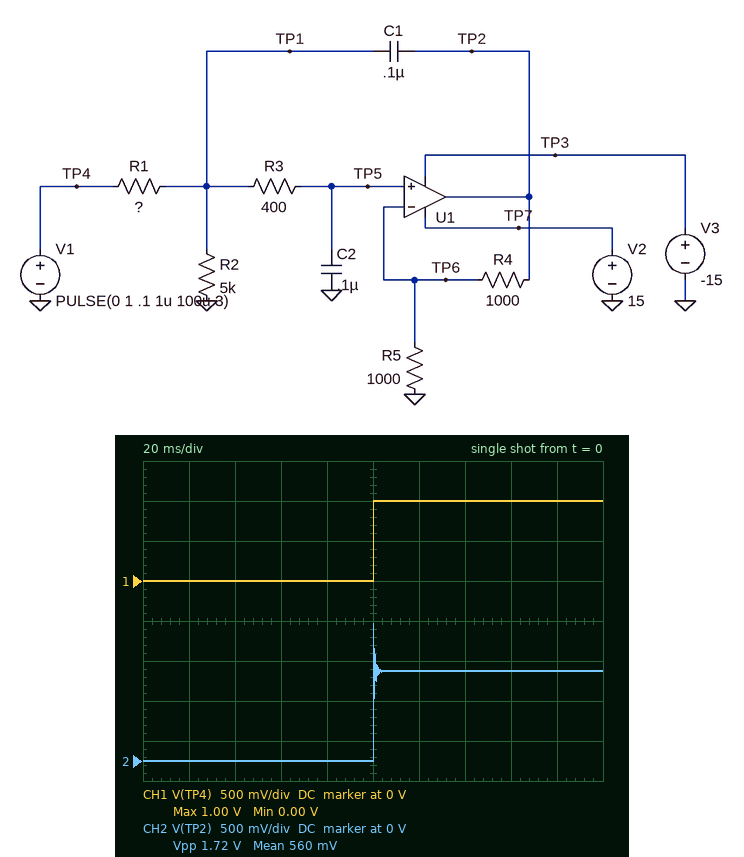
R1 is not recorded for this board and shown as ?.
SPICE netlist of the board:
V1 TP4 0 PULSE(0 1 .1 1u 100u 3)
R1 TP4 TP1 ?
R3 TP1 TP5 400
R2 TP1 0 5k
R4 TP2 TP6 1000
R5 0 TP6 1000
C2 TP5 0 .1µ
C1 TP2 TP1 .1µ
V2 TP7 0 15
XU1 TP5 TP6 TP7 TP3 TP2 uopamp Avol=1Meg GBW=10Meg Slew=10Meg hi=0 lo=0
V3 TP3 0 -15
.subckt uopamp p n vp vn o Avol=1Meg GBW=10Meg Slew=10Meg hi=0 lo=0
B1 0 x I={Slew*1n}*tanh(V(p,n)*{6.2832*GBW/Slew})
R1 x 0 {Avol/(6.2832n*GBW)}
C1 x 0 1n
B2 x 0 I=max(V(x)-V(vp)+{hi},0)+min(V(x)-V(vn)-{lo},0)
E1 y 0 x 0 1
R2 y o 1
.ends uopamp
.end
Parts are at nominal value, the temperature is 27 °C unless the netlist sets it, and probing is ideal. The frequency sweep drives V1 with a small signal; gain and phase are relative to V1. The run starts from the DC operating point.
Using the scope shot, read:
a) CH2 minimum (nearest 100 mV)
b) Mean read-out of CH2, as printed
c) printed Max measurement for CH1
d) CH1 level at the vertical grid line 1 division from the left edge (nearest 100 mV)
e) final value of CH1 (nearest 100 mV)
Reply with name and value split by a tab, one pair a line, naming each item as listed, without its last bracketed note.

CH2 minimum	0 V
Mean read-out of CH2, as printed	560 mV
printed Max measurement for CH1	1.00 V
CH1 level at the vertical grid line 1 division from the left edge	0 V
final value of CH1	1.0 V
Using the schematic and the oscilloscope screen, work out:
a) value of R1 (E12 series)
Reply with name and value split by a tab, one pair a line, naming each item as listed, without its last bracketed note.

value of R1	3.9 kΩ
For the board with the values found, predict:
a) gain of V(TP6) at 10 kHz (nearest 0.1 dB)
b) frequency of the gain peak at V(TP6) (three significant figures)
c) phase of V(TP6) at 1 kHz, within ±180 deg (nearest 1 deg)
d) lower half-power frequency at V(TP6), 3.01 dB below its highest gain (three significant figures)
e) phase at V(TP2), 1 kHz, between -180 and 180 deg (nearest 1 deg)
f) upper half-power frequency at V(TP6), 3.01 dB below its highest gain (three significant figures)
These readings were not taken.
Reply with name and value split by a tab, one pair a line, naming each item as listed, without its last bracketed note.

gain of V(TP6) at 10 kHz	-35.6 dB
frequency of the gain peak at V(TP6)	1.62 kHz
phase of V(TP6) at 1 kHz, within ±180 deg	-21 deg
lower half-power frequency at V(TP6), 3.01 dB below its highest gain	1.19 kHz
phase at V(TP2), 1 kHz, between -180 and 180 deg	-21 deg
upper half-power frequency at V(TP6), 3.01 dB below its highest gain	1.96 kHz
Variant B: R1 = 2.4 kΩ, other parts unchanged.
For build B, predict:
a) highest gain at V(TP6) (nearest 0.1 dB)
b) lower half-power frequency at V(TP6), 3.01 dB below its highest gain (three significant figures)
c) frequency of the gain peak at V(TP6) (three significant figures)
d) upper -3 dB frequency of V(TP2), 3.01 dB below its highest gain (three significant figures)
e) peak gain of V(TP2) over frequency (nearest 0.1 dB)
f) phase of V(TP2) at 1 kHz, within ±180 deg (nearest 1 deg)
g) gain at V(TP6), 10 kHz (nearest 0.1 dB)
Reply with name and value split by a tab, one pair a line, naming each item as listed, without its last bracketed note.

highest gain at V(TP6)	3.0 dB
lower half-power frequency at V(TP6), 3.01 dB below its highest gain	1.24 kHz
frequency of the gain peak at V(TP6)	1.85 kHz
upper -3 dB frequency of V(TP2), 3.01 dB below its highest gain	2.30 kHz
peak gain of V(TP2) over frequency	9.0 dB
phase of V(TP2) at 1 kHz, within ±180 deg	-19 deg
gain at V(TP6), 10 kHz	-31.3 dB
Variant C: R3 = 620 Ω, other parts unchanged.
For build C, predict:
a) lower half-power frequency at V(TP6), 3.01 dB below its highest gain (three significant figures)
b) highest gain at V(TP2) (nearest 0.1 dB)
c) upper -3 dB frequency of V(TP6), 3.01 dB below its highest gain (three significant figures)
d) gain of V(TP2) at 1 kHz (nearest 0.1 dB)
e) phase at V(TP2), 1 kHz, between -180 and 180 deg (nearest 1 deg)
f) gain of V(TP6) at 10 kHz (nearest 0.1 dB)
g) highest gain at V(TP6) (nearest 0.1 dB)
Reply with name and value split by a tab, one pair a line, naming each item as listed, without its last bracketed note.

lower half-power frequency at V(TP6), 3.01 dB below its highest gain	803 Hz
highest gain at V(TP2)	6.8 dB
upper -3 dB frequency of V(TP6), 3.01 dB below its highest gain	1.60 kHz
gain of V(TP2) at 1 kHz	5.4 dB
phase at V(TP2), 1 kHz, between -180 and 180 deg	-40 deg
gain of V(TP6) at 10 kHz	-39.5 dB
highest gain at V(TP6)	0.8 dB
